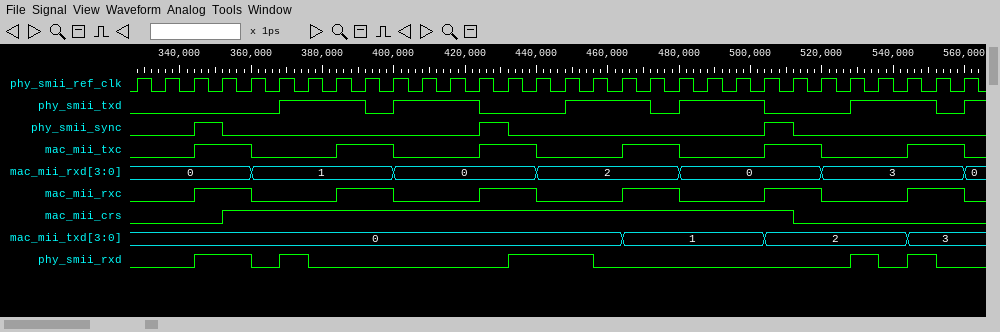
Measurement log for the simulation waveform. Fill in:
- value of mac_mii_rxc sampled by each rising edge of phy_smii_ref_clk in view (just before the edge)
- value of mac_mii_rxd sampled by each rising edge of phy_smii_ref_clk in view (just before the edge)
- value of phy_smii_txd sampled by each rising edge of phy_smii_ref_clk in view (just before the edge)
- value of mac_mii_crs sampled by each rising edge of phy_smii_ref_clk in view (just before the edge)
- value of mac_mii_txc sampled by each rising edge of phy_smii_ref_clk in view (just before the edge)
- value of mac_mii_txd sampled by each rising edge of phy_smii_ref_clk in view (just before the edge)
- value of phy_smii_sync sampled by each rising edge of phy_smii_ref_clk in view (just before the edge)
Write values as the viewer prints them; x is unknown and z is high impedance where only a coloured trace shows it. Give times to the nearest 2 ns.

0 0 0 1 1 0 0 0 1 1 0 0 0 1 1 0 0 0 1 1 0 0 0 1 1 0 0 0 1 1
0, 0, 0, 0, 0, 1, 1, 1, 1, 1, 0, 0, 0, 0, 0, 2, 2, 2, 2, 2, 0, 0, 0, 0, 0, 3, 3, 3, 3, 3
0 0 0 0 0 0 1 1 1 0 1 1 1 0 0 0 1 1 1 0 1 1 1 0 0 0 1 1 1 0
0 0 0 0 1 1 1 1 1 1 1 1 1 1 1 1 1 1 1 1 1 1 1 1 0 0 0 0 0 0
0 0 0 1 1 0 0 0 1 1 0 0 0 1 1 0 0 0 1 1 0 0 0 1 1 0 0 0 1 1
0, 0, 0, 0, 0, 0, 0, 0, 0, 0, 0, 0, 0, 0, 0, 0, 0, 0, 1, 1, 1, 1, 1, 2, 2, 2, 2, 2, 3, 3
0 0 0 1 0 0 0 0 0 0 0 0 0 1 0 0 0 0 0 0 0 0 0 1 0 0 0 0 0 0
